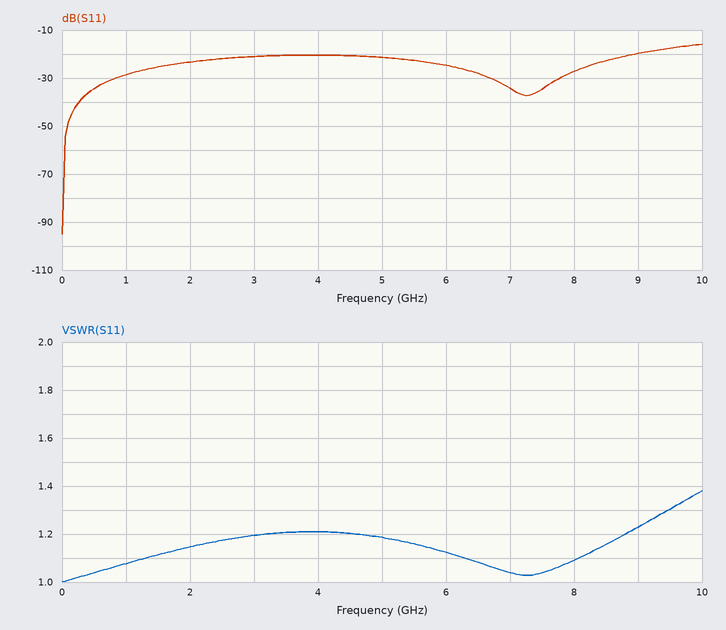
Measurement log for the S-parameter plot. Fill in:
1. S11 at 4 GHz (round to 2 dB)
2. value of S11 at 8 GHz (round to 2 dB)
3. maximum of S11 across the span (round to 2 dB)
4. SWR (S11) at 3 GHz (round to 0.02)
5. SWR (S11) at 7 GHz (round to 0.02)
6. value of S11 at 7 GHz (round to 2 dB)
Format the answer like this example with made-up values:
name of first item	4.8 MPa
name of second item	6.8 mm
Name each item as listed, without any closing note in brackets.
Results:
S11 at 4 GHz	-20 dB
value of S11 at 8 GHz	-28 dB
maximum of S11 across the span	-16 dB
SWR (S11) at 3 GHz	1.20
SWR (S11) at 7 GHz	1.04
value of S11 at 7 GHz	-34 dB
